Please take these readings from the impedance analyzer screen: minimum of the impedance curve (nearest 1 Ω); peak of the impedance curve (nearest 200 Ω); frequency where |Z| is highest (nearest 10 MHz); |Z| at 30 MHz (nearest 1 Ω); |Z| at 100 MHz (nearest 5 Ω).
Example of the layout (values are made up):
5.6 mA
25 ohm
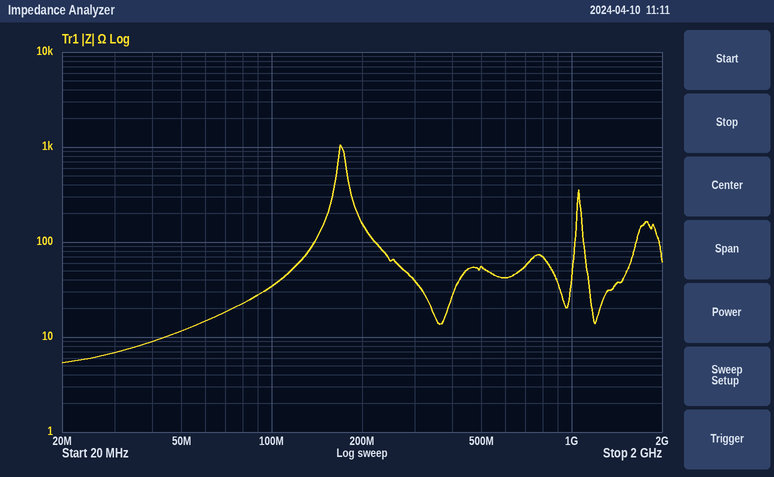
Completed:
5 Ω
1.0 kΩ
170 MHz
7 Ω
35 Ω
